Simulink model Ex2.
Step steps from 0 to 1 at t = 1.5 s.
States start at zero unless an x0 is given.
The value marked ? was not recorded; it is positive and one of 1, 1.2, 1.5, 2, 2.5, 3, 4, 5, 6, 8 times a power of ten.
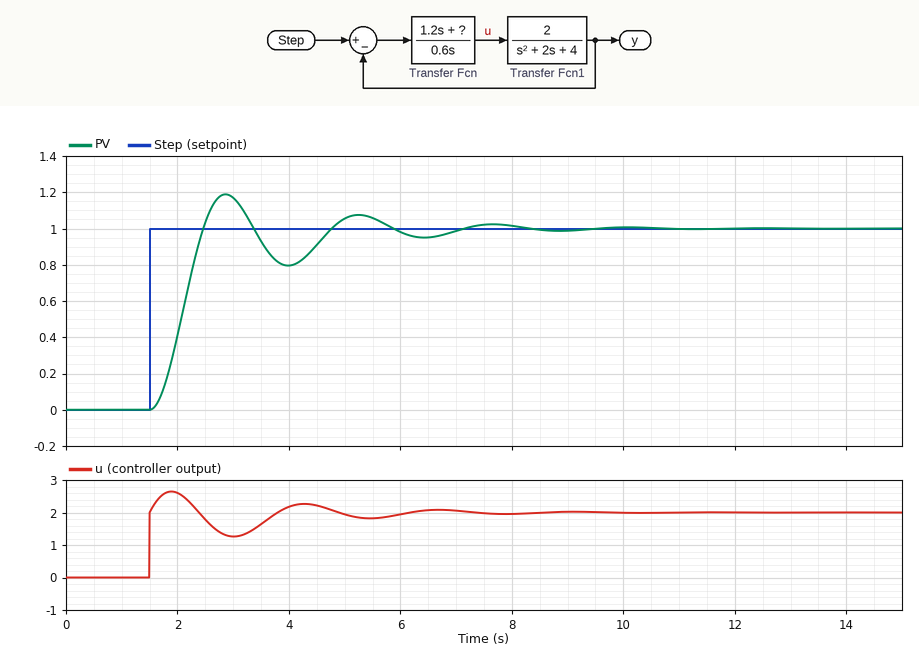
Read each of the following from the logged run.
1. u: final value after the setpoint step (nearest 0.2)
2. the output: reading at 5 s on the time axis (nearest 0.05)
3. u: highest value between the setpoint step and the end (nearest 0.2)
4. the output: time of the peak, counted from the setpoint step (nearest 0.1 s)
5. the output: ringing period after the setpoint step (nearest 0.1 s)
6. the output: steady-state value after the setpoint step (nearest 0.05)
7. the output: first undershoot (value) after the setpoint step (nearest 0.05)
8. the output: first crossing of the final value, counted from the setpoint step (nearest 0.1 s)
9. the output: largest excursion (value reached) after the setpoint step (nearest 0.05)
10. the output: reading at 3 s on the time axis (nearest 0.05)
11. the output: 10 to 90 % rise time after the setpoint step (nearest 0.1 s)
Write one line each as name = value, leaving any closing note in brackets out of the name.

u: final value after the setpoint step = 2.0
the output: reading at 5 s on the time axis = 1.05
u: highest value between the setpoint step and the end = 2.6
the output: time of the peak, counted from the setpoint step = 1.4 s
the output: ringing period after the setpoint step = 2.4 s
the output: steady-state value after the setpoint step = 1.00
the output: first undershoot (value) after the setpoint step = 0.80
the output: first crossing of the final value, counted from the setpoint step = 1.0 s
the output: largest excursion (value reached) after the setpoint step = 1.20
the output: reading at 3 s on the time axis = 1.15
the output: 10 to 90 % rise time after the setpoint step = 0.6 s
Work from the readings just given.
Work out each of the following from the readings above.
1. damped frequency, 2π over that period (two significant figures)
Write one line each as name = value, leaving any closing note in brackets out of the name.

damped frequency, 2π over that period = 2.6 rad/s
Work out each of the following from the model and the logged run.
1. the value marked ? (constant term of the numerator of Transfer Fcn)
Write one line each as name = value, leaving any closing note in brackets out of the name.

the value marked ? = 2
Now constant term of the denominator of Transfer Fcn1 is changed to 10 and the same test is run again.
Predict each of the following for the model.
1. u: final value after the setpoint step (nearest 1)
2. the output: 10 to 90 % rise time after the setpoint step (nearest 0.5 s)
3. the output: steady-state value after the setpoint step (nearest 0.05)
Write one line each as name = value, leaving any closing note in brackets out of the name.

u: final value after the setpoint step = 5
the output: 10 to 90 % rise time after the setpoint step = 4.0 s
the output: steady-state value after the setpoint step = 1.00
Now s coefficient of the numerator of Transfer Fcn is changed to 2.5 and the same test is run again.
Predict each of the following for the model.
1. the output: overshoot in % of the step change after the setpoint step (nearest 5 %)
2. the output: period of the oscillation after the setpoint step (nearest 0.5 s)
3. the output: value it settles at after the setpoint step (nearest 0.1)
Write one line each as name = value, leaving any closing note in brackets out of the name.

the output: overshoot in % of the step change after the setpoint step = 20 %
the output: period of the oscillation after the setpoint step = 2.0 s
the output: value it settles at after the setpoint step = 1.0
